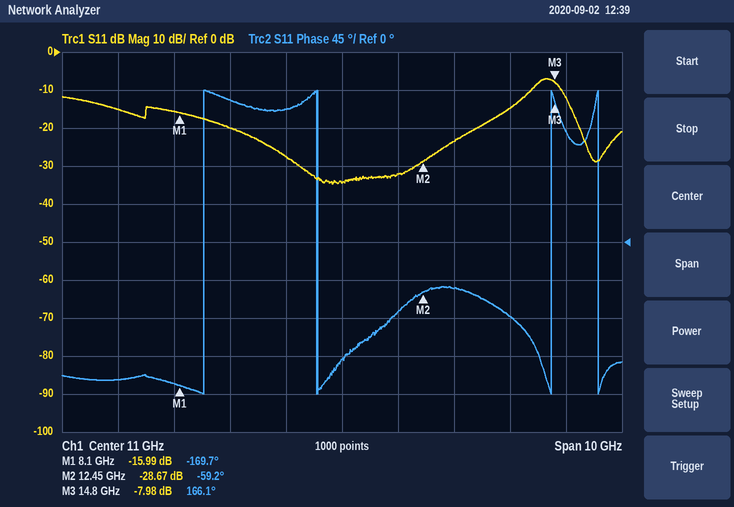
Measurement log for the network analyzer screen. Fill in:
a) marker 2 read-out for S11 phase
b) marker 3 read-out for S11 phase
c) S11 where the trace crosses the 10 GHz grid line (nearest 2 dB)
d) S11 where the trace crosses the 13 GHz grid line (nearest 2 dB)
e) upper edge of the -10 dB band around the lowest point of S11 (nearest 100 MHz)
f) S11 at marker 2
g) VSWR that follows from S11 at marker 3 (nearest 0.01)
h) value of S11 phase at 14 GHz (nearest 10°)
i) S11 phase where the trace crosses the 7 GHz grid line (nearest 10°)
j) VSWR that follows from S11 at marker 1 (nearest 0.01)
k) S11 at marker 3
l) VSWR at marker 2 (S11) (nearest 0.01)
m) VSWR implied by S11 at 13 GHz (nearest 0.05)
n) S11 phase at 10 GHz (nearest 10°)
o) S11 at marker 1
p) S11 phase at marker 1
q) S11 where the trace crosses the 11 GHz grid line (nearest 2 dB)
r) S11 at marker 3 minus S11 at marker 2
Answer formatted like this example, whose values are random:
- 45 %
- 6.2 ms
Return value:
- -59.2°
- 166.1°
- -28 dB
- -24 dB
- 14.4 GHz
- -28.67 dB
- 2.33
- -90°
- -160°
- 1.38
- -7.98 dB
- 1.08
- 1.15
- 160°
- -15.99 dB
- -169.7°
- -34 dB
- 20.69 dB
